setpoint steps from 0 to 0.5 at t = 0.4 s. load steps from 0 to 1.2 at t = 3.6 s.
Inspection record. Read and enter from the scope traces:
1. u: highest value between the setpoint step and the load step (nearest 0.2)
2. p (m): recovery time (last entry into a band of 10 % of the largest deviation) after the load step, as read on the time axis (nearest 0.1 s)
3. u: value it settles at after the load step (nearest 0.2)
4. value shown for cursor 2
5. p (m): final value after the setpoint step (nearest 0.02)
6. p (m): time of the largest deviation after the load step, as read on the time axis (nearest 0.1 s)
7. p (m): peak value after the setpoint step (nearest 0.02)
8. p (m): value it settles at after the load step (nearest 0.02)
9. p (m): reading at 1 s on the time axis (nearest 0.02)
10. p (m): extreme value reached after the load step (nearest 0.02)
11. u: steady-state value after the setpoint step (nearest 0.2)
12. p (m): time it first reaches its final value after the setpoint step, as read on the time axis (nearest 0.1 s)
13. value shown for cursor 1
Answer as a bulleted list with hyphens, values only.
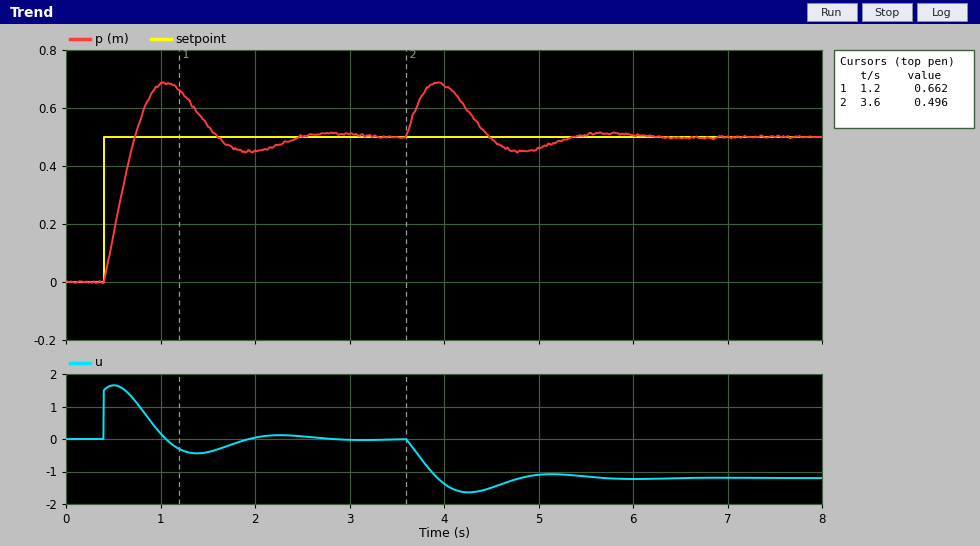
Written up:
- 1.6
- 5.2 s
- -1.2
- 0.496
- 0.50
- 3.9 s
- 0.68
- 0.50
- 0.68
- 0.68
- 0.0
- 0.7 s
- 0.662
